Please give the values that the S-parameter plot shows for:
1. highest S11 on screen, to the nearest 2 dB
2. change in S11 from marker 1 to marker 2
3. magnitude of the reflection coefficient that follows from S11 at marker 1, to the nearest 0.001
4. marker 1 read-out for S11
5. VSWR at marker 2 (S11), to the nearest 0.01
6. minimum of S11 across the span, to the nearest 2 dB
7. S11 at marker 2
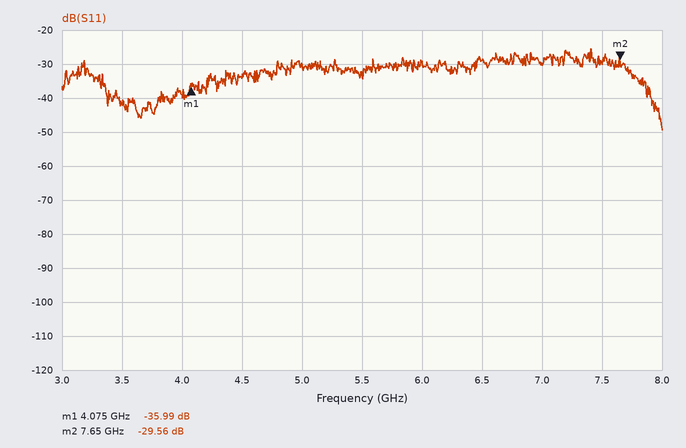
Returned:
-26 dB
6.43 dB
0.016
-35.99 dB
1.07
-50 dB
-29.56 dB
